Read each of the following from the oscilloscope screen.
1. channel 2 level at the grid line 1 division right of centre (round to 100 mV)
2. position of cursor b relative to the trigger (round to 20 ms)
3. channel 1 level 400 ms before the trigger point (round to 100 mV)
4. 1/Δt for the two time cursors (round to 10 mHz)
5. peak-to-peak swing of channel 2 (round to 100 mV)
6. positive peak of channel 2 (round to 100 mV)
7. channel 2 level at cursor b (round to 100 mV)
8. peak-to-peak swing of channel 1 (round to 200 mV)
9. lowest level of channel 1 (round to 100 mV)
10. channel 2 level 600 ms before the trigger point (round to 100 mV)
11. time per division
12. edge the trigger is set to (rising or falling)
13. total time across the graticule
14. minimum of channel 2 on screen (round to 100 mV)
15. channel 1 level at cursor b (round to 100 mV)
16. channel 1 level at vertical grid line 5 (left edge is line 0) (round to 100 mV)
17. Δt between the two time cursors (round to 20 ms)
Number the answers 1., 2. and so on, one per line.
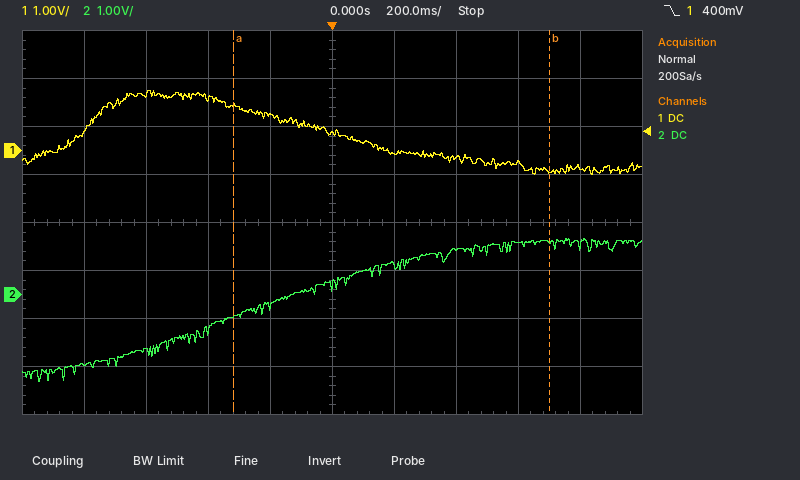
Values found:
1. 600 mV
2. +700 ms
3. 1.1 V
4. 980 mHz
5. 3.0 V
6. 1.2 V
7. 1.1 V
8. 1.8 V
9. -500 mV
10. -1.2 V
11. 200 ms
12. falling
13. 2 s
14. -1.8 V
15. -400 mV
16. 400 mV
17. 1.02 s
